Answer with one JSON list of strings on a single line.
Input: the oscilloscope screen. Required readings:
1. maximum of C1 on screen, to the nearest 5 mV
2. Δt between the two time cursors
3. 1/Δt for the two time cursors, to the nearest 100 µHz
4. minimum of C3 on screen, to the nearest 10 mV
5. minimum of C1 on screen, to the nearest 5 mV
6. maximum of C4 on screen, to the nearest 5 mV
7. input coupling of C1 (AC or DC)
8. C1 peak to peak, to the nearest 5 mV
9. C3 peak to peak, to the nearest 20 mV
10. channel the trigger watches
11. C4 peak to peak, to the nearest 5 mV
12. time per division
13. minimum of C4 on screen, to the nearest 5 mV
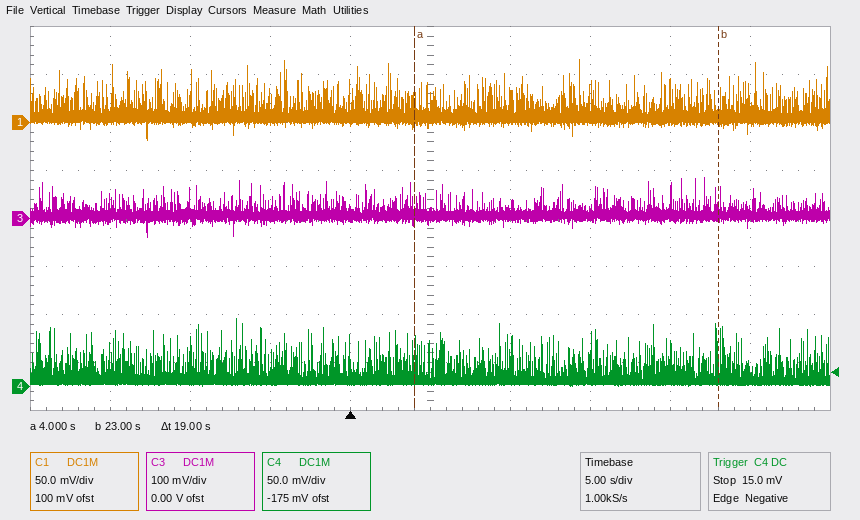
["65 mV", "19 s", "52.6 mHz", "-40 mV", "-20 mV", "70 mV", "DC", "85 mV", "120 mV", "C4", "70 mV", "5 s", "0 mV"]
